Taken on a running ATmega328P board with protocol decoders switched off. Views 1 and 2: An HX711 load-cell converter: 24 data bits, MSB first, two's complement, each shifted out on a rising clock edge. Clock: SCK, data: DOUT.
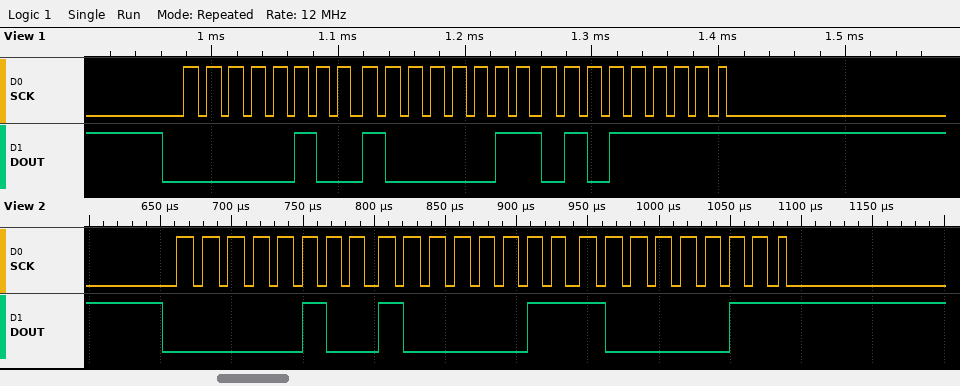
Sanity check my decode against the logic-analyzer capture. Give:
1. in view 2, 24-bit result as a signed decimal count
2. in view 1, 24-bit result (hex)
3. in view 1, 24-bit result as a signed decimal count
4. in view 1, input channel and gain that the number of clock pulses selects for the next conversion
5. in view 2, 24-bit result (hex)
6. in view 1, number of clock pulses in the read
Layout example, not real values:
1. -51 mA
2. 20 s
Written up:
1. 295811
2. 0x04835F
3. 295775
4. channel A, gain 128
5. 0x048383
6. 25
